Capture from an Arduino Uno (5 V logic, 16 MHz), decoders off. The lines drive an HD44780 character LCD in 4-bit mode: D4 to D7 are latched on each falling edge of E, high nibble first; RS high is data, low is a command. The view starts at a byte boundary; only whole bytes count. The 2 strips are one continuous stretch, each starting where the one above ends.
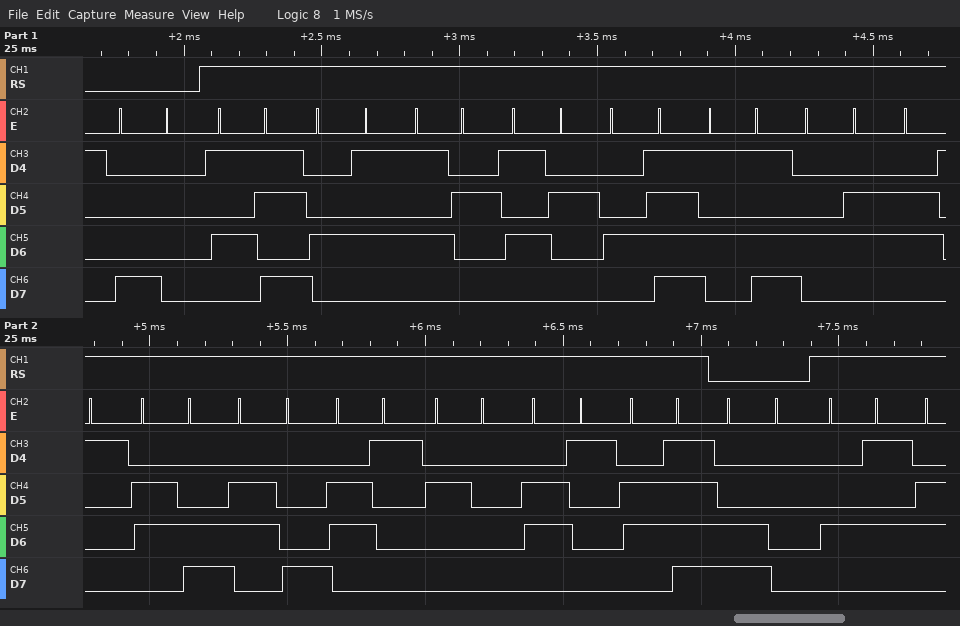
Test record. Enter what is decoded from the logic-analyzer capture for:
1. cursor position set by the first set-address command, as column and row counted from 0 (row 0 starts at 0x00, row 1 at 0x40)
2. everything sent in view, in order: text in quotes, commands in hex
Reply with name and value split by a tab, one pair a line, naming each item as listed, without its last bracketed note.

cursor position set by the first set-address command, as column and row counted from 0	column 0, row 0
everything sent in view, in order: text in quotes, commands in hex	0x80 "[ERRO]Falha ao" 0xC0 "E"
